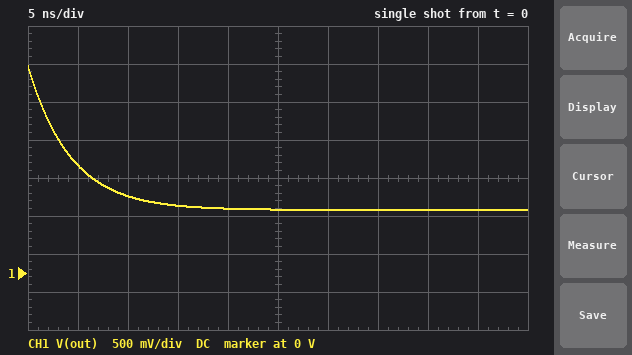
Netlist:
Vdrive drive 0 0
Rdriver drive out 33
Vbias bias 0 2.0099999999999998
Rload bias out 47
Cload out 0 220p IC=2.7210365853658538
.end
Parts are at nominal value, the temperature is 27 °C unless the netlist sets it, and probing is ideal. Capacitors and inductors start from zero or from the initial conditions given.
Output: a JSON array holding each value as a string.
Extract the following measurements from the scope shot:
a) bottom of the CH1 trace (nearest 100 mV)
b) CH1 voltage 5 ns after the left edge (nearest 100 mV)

["800 mV", "1.4 V"]
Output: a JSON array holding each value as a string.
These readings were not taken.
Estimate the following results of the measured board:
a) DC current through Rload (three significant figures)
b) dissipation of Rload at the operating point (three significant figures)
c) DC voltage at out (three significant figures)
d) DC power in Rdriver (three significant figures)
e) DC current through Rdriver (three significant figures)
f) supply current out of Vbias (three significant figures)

["25.1 mA", "29.7 mW", "829 mV", "20.8 mW", "25.1 mA", "25.1 mA"]
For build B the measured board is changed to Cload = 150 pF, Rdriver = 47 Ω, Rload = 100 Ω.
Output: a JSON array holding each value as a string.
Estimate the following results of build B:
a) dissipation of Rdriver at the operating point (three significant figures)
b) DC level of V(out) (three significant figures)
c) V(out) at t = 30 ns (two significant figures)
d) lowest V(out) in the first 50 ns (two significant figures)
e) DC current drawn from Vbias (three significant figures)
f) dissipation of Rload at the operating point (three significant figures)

["8.79 mW", "643 mV", "650 mV", "640 mV", "13.7 mA", "18.7 mW"]
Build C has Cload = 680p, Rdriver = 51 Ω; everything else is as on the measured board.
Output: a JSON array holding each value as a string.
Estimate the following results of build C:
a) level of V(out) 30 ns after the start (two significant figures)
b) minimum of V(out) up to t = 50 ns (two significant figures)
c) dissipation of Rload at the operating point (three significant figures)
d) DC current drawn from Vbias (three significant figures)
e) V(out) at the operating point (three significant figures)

["1.3 V", "1.1 V", "19.8 mW", "20.5 mA", "1.05 V"]
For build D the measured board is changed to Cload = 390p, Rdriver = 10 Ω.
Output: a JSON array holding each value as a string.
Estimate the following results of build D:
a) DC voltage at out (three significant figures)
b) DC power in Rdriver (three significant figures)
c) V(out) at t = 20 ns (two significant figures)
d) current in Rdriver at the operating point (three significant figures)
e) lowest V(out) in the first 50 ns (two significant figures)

["353 mV", "12.4 mW", "360 mV", "35.3 mA", "350 mV"]
